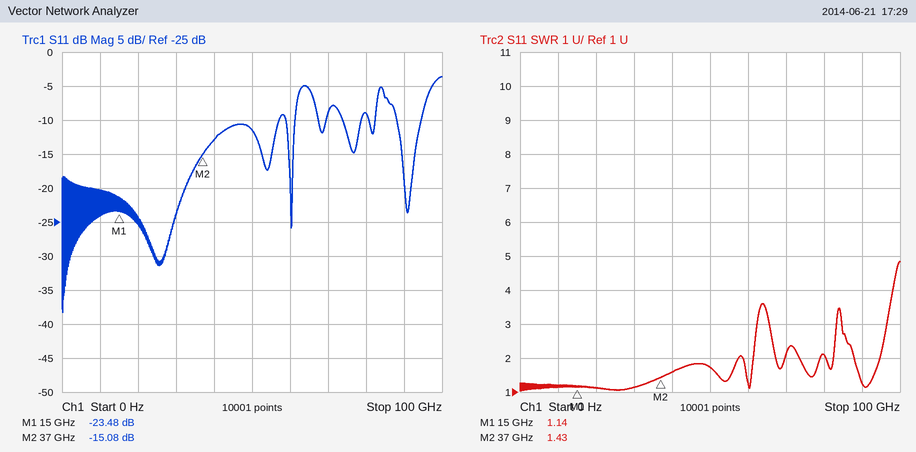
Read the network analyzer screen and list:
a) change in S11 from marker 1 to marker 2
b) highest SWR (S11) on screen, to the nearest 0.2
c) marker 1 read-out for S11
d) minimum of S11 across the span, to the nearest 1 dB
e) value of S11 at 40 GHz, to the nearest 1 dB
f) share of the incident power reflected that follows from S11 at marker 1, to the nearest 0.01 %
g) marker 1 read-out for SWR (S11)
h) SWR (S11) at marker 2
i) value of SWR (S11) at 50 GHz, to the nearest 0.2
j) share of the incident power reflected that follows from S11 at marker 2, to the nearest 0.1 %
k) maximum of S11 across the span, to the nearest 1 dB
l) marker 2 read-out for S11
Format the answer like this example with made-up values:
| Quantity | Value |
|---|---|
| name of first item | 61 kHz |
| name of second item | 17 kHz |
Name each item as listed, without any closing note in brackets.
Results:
| Quantity | Value |
|---|---|
| change in S11 from marker 1 to marker 2 | 8.40 dB |
| highest SWR (S11) on screen, to the nearest 0.2 | 4.8 |
| marker 1 read-out for S11 | -23.48 dB |
| minimum of S11 across the span, to the nearest 1 dB | -38 dB |
| value of S11 at 40 GHz, to the nearest 1 dB | -13 dB |
| share of the incident power reflected that follows from S11 at marker 1, to the nearest 0.01 % | 0.45 % |
| marker 1 read-out for SWR | 1.14 |
| SWR (S11) at marker 2 | 1.43 |
| value of SWR (S11) at 50 GHz, to the nearest 0.2 | 1.8 |
| share of the incident power reflected that follows from S11 at marker 2, to the nearest 0.1 % | 3.1 % |
| maximum of S11 across the span, to the nearest 1 dB | -4 dB |
| marker 2 read-out for S11 | -15.08 dB |
